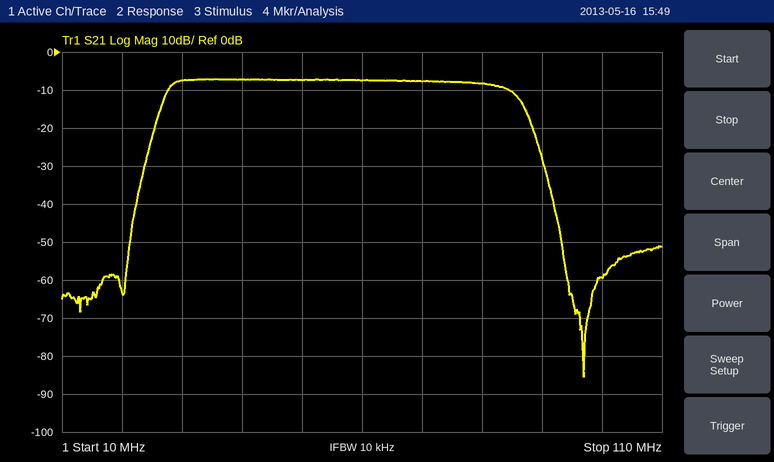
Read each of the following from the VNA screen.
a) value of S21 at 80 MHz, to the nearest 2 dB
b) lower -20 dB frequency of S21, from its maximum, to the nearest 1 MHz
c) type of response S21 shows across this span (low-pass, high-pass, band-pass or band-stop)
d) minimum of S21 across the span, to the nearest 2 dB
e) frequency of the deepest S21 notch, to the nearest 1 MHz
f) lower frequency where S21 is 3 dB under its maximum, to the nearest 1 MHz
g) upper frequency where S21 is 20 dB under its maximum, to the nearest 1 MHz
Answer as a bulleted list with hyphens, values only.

- -8 dB
- 24 MHz
- band-pass
- -86 dB
- 97 MHz
- 28 MHz
- 90 MHz
